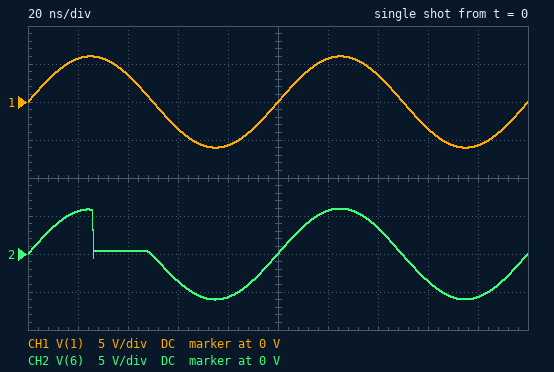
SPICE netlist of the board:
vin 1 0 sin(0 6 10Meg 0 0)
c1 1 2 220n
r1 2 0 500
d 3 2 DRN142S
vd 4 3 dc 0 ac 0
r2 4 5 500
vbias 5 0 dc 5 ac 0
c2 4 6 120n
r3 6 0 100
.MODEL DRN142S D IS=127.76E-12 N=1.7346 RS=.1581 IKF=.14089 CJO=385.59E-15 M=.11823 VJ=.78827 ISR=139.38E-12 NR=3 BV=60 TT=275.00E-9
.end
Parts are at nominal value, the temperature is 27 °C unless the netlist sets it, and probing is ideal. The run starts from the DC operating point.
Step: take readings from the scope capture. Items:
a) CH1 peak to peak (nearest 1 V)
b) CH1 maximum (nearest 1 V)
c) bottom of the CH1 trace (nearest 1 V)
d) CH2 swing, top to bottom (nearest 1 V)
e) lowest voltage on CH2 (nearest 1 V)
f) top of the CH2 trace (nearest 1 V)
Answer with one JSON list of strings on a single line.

["12 V", "6 V", "-6 V", "12 V", "-6 V", "6 V"]
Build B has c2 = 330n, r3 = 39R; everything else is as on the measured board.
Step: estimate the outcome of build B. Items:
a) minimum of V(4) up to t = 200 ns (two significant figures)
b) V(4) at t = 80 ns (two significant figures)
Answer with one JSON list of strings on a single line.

["-3.0 V", "-2.7 V"]
